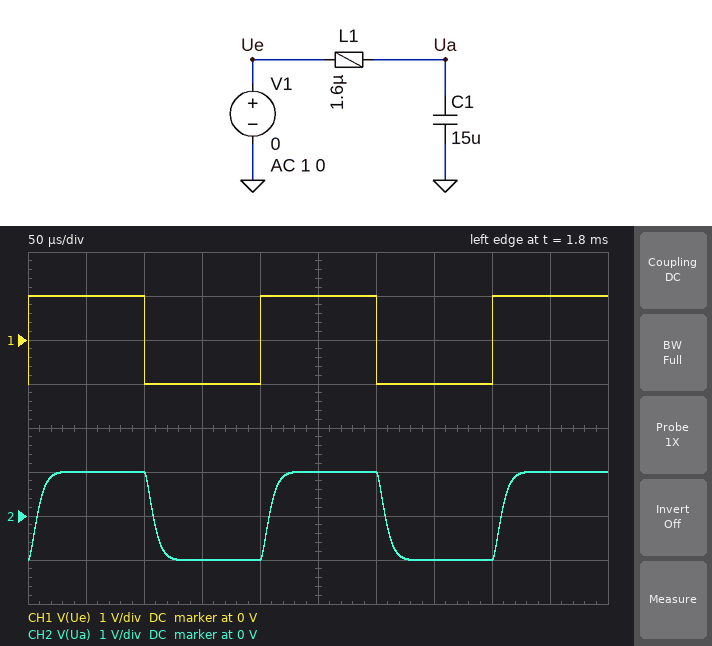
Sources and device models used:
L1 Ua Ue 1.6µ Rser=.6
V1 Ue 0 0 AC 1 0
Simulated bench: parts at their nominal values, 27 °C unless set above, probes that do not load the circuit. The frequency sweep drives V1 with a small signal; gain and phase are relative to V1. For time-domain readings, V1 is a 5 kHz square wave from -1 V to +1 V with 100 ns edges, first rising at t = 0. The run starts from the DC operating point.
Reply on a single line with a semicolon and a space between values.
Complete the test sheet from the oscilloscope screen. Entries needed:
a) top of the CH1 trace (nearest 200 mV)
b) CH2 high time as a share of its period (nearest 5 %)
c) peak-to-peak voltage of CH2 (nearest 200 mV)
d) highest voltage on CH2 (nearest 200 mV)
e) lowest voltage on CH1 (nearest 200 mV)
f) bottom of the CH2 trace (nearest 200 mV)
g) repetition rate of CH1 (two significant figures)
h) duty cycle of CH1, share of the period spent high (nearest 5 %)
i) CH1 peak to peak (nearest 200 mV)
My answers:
1.0 V; 50 %; 2.0 V; 1.0 V; -1.0 V; -1.0 V; 5.0 kHz; 50 %; 2.0 V
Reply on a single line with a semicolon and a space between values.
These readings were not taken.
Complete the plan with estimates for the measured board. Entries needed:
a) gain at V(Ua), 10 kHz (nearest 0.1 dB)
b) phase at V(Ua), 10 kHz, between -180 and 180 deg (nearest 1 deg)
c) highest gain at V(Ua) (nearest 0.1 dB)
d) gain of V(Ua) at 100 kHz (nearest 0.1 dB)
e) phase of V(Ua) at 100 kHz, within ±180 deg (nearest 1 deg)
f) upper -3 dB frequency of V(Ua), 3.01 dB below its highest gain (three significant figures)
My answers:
-0.6 dB; -32 deg; 0 dB; -20.2 dB; -146 deg; 23.6 kHz
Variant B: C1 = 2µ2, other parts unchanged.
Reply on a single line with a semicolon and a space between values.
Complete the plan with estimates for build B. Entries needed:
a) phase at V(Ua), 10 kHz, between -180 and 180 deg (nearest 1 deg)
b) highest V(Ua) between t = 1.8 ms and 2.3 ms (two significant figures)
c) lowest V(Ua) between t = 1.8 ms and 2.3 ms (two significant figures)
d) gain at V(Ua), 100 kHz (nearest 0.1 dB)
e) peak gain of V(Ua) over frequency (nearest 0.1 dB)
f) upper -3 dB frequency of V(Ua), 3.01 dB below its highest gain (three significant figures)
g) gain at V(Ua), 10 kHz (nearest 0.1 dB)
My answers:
-5 deg; 1.6 V; -1.6 V; 0.8 dB; 3.6 dB; 101 kHz; 0.1 dB
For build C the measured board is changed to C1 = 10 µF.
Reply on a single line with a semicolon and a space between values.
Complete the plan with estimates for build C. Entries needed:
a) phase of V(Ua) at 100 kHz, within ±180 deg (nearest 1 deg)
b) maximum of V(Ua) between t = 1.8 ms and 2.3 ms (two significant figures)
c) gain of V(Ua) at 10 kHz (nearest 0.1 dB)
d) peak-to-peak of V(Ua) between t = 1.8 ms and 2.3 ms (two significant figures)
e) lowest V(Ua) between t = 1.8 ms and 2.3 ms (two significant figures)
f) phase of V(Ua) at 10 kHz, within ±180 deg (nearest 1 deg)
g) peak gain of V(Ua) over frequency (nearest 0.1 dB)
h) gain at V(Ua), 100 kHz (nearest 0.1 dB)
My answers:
-145 deg; 1.1 V; -0.1 dB; 2.1 V; -1.1 V; -22 deg; 0 dB; -16.3 dB
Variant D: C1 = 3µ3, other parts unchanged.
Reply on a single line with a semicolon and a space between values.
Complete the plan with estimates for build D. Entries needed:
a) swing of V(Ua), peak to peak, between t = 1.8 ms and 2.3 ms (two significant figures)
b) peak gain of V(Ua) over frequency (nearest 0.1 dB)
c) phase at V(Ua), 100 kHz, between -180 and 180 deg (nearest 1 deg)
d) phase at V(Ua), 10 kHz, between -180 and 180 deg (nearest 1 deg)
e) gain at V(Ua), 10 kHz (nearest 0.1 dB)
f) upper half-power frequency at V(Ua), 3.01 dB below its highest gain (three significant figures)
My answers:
2.9 V; 2.2 dB; -131 deg; -7 deg; 0.1 dB; 82.1 kHz
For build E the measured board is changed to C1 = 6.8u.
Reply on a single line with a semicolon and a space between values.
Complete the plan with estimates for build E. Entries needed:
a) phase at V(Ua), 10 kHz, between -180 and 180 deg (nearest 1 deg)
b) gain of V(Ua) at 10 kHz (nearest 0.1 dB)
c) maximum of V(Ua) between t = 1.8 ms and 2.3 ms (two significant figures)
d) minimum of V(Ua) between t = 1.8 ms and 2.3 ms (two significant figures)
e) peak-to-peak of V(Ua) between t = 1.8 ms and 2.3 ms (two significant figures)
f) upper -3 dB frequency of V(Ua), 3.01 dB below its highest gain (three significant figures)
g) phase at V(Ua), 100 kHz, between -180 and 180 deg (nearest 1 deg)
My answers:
-15 deg; 0.1 dB; 1.2 V; -1.2 V; 2.3 V; 53.0 kHz; -142 deg
